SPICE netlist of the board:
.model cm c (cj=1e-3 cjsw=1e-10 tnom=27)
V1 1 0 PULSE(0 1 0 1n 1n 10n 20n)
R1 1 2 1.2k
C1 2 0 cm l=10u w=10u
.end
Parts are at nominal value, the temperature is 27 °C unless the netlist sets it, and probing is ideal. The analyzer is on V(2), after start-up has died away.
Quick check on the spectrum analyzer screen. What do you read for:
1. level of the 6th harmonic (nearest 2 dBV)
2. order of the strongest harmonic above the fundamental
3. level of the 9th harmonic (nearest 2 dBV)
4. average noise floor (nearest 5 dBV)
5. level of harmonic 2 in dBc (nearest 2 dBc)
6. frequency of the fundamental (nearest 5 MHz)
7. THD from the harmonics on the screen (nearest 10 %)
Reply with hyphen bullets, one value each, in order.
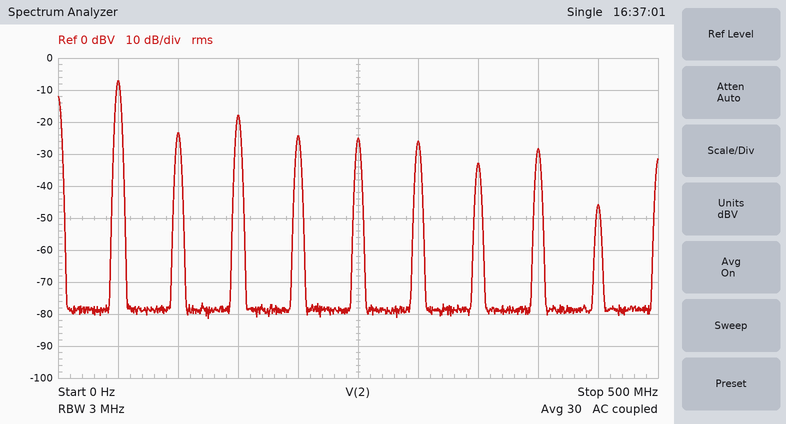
- -26 dBV
- 3
- -46 dBV
- -80 dBV
- -16 dBc
- 50 MHz
- 40 %
